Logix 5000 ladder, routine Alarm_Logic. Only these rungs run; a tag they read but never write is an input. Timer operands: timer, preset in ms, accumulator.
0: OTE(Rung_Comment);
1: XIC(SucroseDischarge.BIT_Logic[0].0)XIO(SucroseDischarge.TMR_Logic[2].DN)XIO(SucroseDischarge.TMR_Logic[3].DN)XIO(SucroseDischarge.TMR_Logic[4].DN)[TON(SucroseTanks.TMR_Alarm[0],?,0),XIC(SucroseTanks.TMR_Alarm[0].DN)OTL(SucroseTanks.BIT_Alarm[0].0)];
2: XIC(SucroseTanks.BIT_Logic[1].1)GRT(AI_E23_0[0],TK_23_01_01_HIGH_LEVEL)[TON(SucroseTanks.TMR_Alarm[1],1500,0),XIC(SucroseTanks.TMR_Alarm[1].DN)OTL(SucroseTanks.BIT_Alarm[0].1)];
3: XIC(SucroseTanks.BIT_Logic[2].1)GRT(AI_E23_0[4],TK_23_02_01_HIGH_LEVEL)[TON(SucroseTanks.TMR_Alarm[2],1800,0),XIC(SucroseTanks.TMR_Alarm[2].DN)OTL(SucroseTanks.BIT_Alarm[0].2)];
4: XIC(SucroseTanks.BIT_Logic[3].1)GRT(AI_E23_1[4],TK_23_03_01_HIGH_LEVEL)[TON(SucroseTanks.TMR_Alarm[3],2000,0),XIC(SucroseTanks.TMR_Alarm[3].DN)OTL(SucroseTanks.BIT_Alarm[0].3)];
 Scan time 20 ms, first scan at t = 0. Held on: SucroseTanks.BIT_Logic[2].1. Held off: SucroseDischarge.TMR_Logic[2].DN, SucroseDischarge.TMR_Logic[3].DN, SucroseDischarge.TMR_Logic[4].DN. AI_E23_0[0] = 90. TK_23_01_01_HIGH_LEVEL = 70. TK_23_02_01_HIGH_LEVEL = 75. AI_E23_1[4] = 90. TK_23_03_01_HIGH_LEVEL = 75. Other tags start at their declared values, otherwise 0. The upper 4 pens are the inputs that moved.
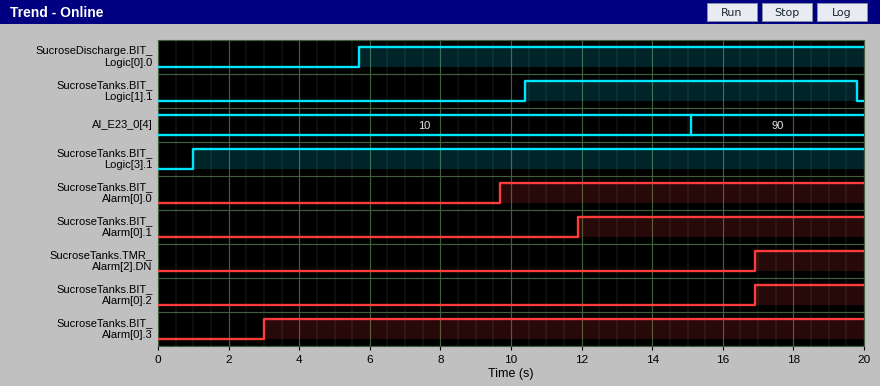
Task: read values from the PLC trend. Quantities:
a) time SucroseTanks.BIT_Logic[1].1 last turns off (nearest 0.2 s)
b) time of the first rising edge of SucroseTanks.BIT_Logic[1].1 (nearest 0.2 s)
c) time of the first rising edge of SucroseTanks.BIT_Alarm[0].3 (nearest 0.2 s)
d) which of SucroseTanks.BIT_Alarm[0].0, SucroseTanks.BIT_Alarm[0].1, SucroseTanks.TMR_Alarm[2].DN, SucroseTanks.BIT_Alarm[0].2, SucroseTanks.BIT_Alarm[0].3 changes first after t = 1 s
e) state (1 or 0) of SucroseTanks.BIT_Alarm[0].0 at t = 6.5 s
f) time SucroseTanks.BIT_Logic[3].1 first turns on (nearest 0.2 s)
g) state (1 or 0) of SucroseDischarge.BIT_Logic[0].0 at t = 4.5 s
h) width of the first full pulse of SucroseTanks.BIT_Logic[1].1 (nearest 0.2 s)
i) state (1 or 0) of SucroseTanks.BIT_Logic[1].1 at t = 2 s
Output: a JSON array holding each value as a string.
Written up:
["19.8 s", "10.4 s", "3.0 s", "SucroseTanks.BIT_Alarm[0].3", "0", "1.0 s", "0", "9.4 s", "0"]
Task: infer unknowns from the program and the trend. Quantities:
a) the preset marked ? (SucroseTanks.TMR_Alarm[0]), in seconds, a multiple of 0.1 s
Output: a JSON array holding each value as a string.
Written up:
["4.0 s"]
